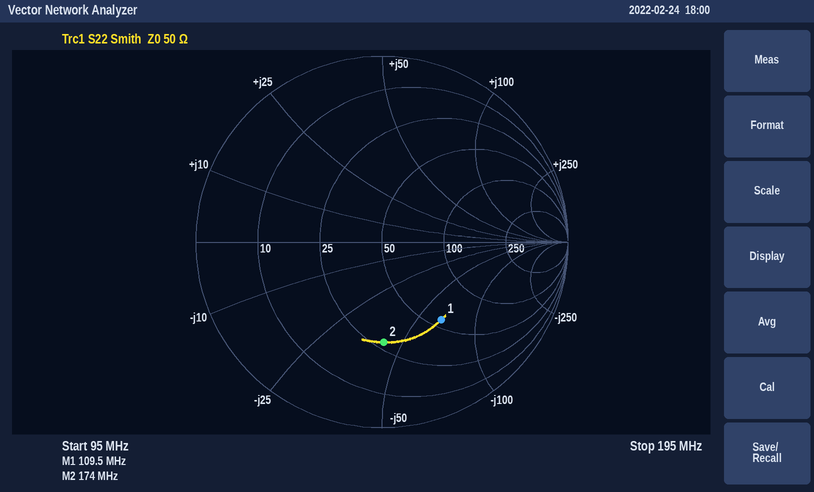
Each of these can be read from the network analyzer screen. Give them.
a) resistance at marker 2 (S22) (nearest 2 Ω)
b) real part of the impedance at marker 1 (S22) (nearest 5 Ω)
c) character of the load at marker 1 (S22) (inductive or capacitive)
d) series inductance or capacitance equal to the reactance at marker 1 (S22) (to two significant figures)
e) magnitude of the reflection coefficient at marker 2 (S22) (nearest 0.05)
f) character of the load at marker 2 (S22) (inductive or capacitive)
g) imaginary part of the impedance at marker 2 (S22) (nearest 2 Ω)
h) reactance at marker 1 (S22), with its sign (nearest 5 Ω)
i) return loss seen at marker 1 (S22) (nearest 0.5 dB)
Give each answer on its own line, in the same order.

28 Ω
55 Ω
capacitive
22 pF
0.55
capacitive
-42 Ω
-65 Ω
5.5 dB
